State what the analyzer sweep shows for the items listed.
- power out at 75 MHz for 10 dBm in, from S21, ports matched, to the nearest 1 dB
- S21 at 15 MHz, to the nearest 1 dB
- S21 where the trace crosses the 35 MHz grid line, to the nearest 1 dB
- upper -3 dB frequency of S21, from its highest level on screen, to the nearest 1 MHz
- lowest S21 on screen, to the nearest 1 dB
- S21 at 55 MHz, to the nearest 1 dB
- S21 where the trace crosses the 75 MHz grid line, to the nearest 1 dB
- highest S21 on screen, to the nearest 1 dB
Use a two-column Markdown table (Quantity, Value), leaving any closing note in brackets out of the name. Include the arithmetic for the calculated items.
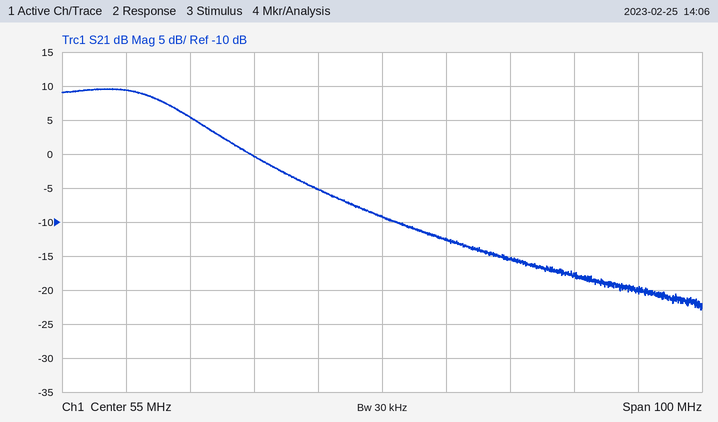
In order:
| Quantity | Value |
|---|---|
| power out at 75 MHz for 10 dBm in, from S21, ports matched, to the nearest 1 dB | 10 dBm + (-15 dB) = -5 dBm |
| S21 at 15 MHz, to the nearest 1 dB | 9 dB |
| S21 where the trace crosses the 35 MHz grid line, to the nearest 1 dB | 0 dB |
| upper -3 dB frequency of S21, from its highest level on screen, to the nearest 1 MHz | 23 MHz |
| lowest S21 on screen, to the nearest 1 dB | -23 dB |
| S21 at 55 MHz, to the nearest 1 dB | -9 dB |
| S21 where the trace crosses the 75 MHz grid line, to the nearest 1 dB | -15 dB |
| highest S21 on screen, to the nearest 1 dB | 10 dB |
